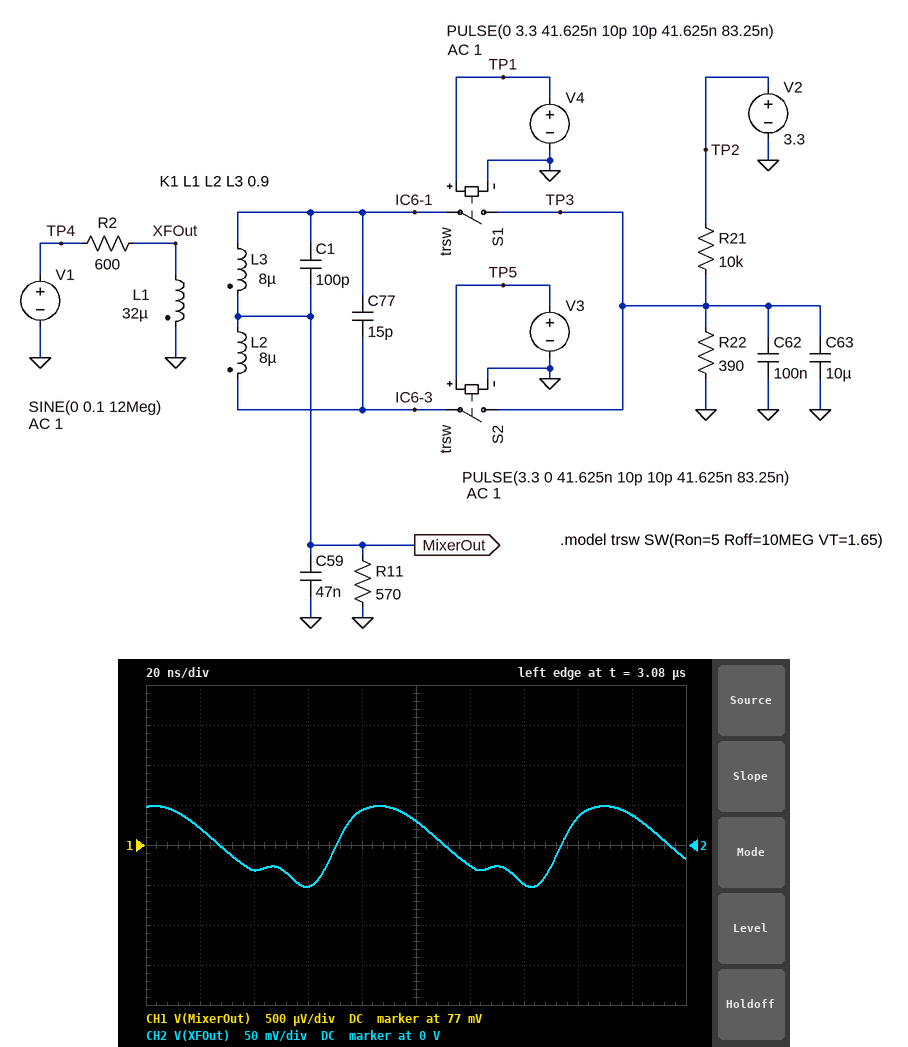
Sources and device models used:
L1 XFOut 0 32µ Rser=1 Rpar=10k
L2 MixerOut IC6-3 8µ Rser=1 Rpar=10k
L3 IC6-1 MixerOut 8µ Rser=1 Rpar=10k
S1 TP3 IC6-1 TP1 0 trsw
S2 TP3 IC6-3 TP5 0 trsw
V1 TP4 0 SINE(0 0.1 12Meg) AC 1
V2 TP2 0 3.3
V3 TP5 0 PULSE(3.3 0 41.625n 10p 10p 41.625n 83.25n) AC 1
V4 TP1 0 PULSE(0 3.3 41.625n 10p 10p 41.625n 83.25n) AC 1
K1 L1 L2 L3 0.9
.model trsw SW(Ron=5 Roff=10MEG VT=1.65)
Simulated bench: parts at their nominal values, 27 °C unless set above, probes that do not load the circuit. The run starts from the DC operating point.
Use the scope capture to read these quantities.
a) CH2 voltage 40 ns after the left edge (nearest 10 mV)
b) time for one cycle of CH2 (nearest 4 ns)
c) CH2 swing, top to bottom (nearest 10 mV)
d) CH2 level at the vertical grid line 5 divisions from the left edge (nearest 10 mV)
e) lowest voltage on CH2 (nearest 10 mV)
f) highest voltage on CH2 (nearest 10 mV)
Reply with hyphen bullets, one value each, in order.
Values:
- -30 mV
- 84 ns
- 100 mV
- 30 mV
- -50 mV
- 50 mV
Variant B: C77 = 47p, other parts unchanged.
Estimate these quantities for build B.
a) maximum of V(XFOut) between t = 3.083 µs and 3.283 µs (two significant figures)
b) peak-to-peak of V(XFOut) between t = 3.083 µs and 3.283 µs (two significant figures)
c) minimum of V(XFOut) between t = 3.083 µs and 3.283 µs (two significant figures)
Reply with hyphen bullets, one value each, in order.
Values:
- 37 mV
- 71 mV
- -34 mV
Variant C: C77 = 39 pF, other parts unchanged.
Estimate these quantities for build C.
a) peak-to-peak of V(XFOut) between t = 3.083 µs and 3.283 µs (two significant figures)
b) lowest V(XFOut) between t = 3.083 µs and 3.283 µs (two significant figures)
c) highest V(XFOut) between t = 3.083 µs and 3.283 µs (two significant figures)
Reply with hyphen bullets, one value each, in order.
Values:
- 71 mV
- -31 mV
- 40 mV
